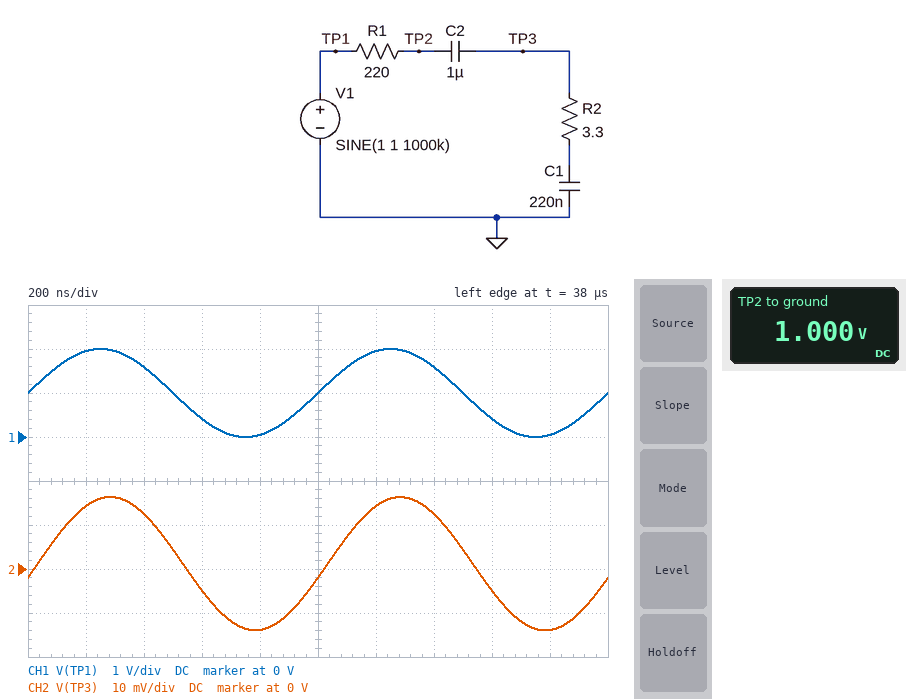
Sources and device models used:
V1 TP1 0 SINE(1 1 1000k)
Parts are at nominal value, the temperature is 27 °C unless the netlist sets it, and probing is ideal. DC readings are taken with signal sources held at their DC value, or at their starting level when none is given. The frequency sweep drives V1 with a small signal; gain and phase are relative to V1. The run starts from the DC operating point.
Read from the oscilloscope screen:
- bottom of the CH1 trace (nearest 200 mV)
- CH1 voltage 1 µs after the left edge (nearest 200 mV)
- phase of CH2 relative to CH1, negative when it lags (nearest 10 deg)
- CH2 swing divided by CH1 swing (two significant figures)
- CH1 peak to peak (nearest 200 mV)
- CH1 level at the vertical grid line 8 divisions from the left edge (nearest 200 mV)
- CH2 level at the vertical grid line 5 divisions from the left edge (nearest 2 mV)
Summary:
0 V
1.0 V
-10 deg
0.015
2.0 V
400 mV
-2 mV
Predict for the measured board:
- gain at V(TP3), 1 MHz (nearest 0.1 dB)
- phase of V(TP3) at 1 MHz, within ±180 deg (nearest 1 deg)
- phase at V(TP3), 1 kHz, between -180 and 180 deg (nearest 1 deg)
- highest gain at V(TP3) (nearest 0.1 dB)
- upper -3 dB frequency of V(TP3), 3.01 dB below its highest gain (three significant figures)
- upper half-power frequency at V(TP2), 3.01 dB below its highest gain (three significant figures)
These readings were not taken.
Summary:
-36.4 dB
-12 deg
-14 deg
-1.7 dB
3.95 kHz
3.95 kHz
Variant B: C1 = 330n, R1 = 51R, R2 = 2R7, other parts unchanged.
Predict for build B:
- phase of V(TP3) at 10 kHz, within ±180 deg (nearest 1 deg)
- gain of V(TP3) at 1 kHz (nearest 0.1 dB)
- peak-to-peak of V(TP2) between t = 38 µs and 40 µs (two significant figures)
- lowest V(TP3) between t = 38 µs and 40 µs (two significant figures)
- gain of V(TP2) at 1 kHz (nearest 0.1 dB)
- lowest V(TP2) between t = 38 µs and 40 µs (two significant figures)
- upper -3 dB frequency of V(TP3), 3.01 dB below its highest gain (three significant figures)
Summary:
-37 deg
-2.5 dB
100 mV
-51 mV
0 dB
950 mV
12.0 kHz
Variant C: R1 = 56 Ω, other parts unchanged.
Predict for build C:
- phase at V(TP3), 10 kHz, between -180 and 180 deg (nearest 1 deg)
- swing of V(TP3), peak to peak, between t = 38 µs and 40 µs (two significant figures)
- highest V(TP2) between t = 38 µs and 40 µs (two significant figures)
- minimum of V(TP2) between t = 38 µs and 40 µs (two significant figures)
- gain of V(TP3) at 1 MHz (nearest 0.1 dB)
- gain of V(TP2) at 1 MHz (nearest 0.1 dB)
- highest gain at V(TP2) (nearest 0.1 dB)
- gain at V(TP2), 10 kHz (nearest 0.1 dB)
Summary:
-31 deg
110 mV
1.1 V
940 mV
-24.9 dB
-24.8 dB
0 dB
-1.6 dB
